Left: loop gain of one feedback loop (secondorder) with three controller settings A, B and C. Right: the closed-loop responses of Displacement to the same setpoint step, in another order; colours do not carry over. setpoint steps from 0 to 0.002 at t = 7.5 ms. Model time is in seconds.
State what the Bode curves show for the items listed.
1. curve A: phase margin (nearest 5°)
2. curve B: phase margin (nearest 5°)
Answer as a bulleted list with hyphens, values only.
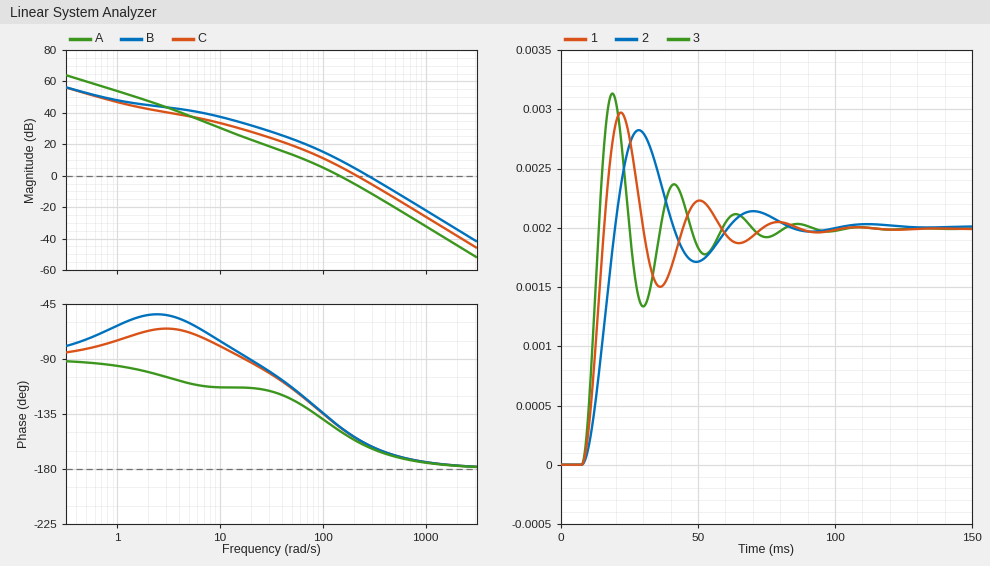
- 30°
- 20°
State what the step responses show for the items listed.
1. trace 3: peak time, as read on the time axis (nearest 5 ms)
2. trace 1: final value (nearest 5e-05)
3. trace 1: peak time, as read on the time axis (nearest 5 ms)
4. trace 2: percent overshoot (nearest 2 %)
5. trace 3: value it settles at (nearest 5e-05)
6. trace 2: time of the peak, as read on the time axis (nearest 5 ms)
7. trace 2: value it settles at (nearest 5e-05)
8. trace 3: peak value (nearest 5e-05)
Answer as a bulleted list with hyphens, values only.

- 20 ms
- 0.00200
- 20 ms
- 42 %
- 0.00200
- 30 ms
- 0.00200
- 0.00315
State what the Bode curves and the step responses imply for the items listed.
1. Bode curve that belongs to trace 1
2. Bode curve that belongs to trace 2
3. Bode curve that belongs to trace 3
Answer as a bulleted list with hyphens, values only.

- C
- A
- B
